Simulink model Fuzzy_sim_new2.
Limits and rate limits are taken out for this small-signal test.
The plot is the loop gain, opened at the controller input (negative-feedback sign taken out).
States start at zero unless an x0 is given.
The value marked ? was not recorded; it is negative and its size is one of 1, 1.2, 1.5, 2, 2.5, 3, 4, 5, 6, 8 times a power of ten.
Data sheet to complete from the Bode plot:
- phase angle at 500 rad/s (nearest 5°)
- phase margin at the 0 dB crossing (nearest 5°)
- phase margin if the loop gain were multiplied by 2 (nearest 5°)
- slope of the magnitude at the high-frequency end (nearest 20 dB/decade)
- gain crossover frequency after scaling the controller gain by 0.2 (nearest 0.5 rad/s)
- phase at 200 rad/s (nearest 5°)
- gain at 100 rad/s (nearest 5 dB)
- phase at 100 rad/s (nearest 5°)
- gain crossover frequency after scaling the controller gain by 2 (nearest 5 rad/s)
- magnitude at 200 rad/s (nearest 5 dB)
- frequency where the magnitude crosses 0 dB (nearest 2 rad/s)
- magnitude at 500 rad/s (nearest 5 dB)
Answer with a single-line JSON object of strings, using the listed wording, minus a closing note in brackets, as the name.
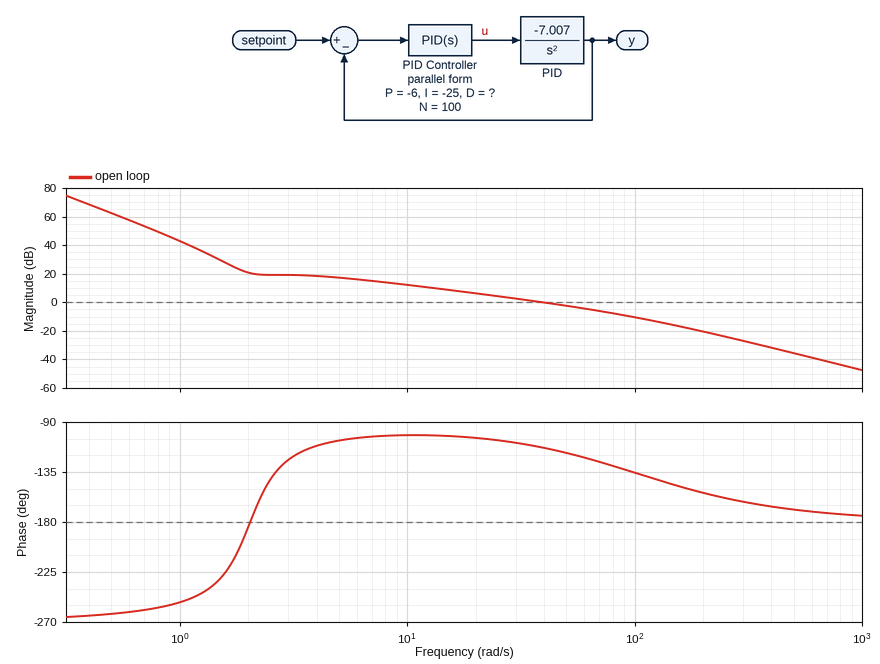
{"phase angle at 500 rad/s": "-170°", "phase margin at the 0 dB crossing": "65°", "phase margin if the loop gain were multiplied by 2": "55°", "slope of the magnitude at the high-frequency end": "-40 dB/decade", "gain crossover frequency after scaling the controller gain by 0.2": "8.0 rad/s", "phase at 200 rad/s": "-155°", "gain at 100 rad/s": "-10 dB", "phase at 100 rad/s": "-135°", "gain crossover frequency after scaling the controller gain by 2": "70 rad/s", "magnitude at 200 rad/s": "-20 dB", "frequency where the magnitude crosses 0 dB": "40 rad/s", "magnitude at 500 rad/s": "-35 dB"}
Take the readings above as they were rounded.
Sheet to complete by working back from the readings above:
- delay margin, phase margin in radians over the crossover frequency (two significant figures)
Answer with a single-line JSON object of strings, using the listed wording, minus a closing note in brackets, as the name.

{"delay margin, phase margin in radians over the crossover frequency": "0.028 s"}
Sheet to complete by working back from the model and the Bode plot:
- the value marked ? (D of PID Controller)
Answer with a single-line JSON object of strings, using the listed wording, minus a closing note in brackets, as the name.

{"the value marked ?": "-6"}
